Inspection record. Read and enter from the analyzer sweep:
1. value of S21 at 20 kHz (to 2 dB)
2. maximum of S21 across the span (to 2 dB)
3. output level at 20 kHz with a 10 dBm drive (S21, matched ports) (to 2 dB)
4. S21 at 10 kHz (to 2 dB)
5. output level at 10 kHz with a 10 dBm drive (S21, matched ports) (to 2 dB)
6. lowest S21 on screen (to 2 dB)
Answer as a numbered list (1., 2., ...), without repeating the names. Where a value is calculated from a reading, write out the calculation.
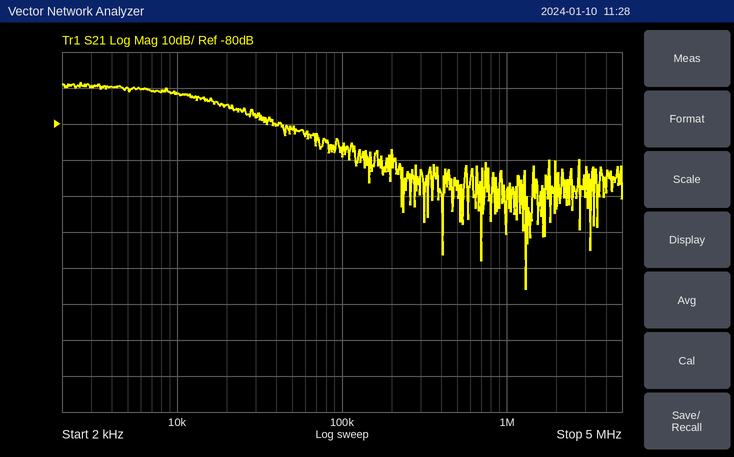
1. -74 dB
2. -68 dB
3. 10 dBm + (-74 dB) = -64 dBm
4. -72 dB
5. 10 dBm + (-72 dB) = -62 dBm
6. -126 dB
